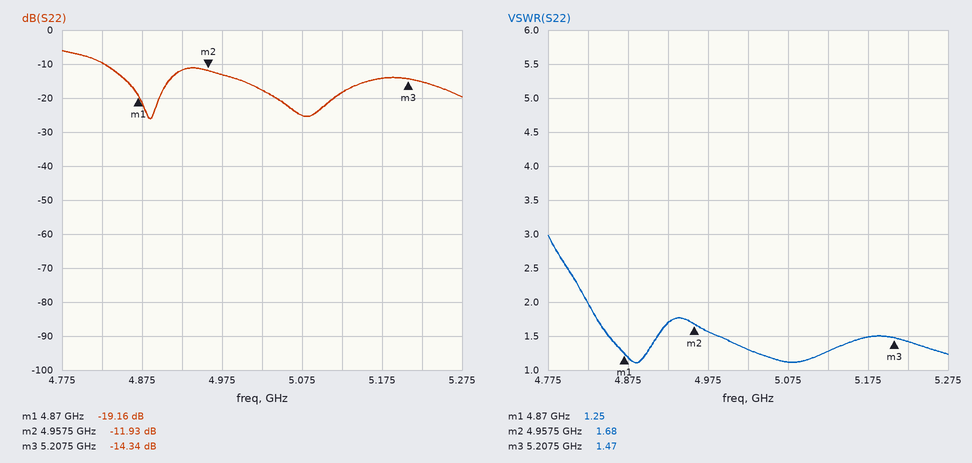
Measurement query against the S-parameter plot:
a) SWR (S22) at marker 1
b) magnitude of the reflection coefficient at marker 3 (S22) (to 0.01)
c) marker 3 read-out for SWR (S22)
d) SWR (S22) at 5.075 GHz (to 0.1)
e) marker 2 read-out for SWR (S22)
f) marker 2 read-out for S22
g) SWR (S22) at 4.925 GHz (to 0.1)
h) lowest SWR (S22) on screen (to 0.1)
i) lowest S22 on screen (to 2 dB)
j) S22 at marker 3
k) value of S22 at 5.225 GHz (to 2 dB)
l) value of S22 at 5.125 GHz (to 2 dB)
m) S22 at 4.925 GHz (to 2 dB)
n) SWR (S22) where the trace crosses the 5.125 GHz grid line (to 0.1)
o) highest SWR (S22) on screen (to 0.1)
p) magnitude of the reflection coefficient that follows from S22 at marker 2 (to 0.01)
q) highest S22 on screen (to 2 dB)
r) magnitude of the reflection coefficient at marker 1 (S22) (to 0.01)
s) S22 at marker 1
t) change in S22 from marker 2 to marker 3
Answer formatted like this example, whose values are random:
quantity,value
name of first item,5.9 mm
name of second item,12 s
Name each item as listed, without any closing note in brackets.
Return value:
quantity,value
SWR (S22) at marker 1,1.25
magnitude of the reflection coefficient at marker 3 (S22),0.19
marker 3 read-out for SWR,1.47
SWR (S22) at 5.075 GHz,1.1
marker 2 read-out for SWR,1.68
marker 2 read-out for S22,-11.93 dB
SWR (S22) at 4.925 GHz,1.7
lowest SWR (S22) on screen,1.1
lowest S22 on screen,-26 dB
S22 at marker 3,-14.34 dB
value of S22 at 5.225 GHz,-16 dB
value of S22 at 5.125 GHz,-18 dB
S22 at 4.925 GHz,-12 dB
SWR (S22) where the trace crosses the 5.125 GHz grid line,1.3
highest SWR (S22) on screen,3.0
magnitude of the reflection coefficient that follows from S22 at marker 2,0.25
highest S22 on screen,-6 dB
magnitude of the reflection coefficient at marker 1 (S22),0.11
S22 at marker 1,-19.16 dB
change in S22 from marker 2 to marker 3,-2.41 dB
